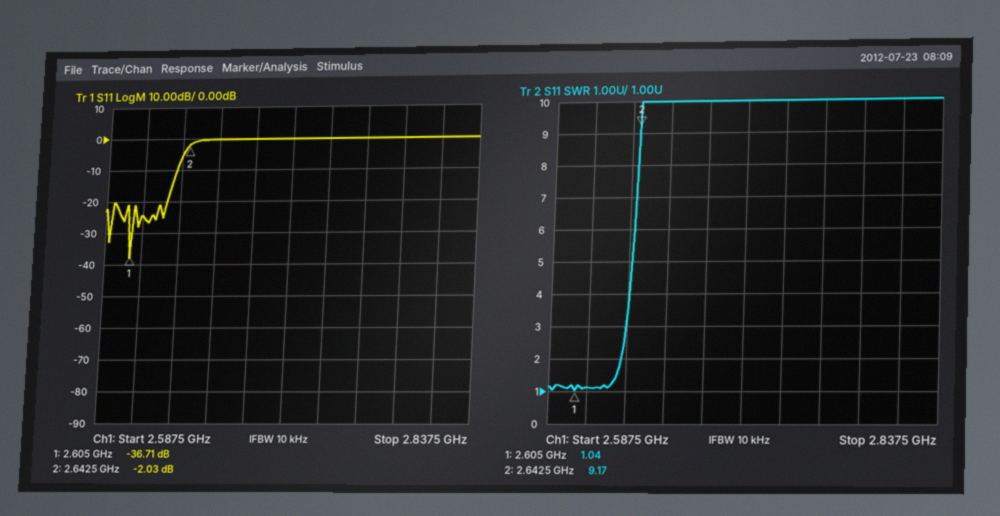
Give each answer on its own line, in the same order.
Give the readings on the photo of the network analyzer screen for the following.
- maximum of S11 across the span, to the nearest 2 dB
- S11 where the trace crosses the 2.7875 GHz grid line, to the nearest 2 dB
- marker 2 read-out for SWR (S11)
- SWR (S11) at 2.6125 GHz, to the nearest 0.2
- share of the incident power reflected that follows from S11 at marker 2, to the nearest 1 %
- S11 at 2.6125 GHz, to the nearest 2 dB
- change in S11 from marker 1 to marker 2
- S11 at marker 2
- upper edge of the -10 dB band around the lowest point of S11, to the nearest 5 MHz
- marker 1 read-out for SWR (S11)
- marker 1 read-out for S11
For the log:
0 dB
0 dB
9.17
1.2
63 %
-24 dB
34.68 dB
-2.03 dB
2.635 GHz
1.04
-36.71 dB
